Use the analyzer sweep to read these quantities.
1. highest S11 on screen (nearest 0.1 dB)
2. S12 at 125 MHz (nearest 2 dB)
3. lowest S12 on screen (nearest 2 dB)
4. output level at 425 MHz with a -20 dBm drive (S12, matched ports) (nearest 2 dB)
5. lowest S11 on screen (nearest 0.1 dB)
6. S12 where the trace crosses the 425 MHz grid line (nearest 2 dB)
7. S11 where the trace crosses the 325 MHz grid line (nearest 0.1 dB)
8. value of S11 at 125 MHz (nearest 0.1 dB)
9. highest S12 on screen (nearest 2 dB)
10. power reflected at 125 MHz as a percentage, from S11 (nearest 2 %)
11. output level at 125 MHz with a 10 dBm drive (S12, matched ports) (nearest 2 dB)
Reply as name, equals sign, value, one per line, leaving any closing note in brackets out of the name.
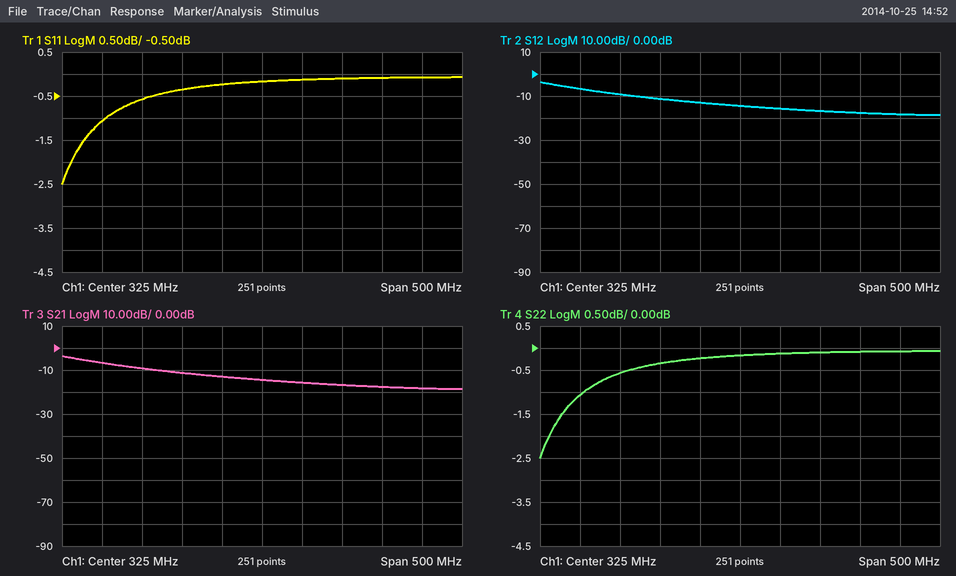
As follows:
highest S11 on screen = -0.1 dB
S12 at 125 MHz = -6 dB
lowest S12 on screen = -18 dB
output level at 425 MHz with a -20 dBm drive (S12, matched ports) = -36 dBm
lowest S11 on screen = -2.5 dB
S12 where the trace crosses the 425 MHz grid line = -16 dB
S11 where the trace crosses the 325 MHz grid line = -0.2 dB
value of S11 at 125 MHz = -1.1 dB
highest S12 on screen = -4 dB
power reflected at 125 MHz as a percentage, from S11 = 78 %
output level at 125 MHz with a 10 dBm drive (S12, matched ports) = 4 dBm
